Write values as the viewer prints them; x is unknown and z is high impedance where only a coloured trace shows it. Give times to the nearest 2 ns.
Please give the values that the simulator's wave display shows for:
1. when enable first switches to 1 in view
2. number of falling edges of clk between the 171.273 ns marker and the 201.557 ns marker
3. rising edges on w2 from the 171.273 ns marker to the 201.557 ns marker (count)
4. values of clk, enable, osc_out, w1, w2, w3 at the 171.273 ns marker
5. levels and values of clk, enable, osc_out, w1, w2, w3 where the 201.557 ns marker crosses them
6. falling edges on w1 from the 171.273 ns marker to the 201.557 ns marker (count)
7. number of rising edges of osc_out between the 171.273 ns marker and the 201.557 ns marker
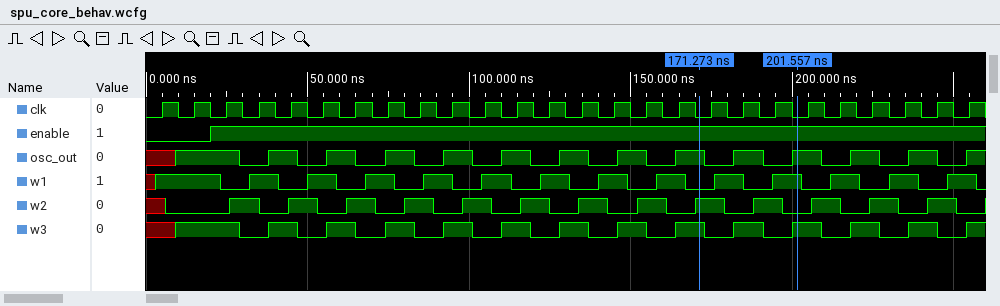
20 ns
3
1
clk=0, enable=1, osc_out=1, w1=0, w2=1, w3=1
clk=0, enable=1, osc_out=1, w1=1, w2=0, w3=1
1
2
